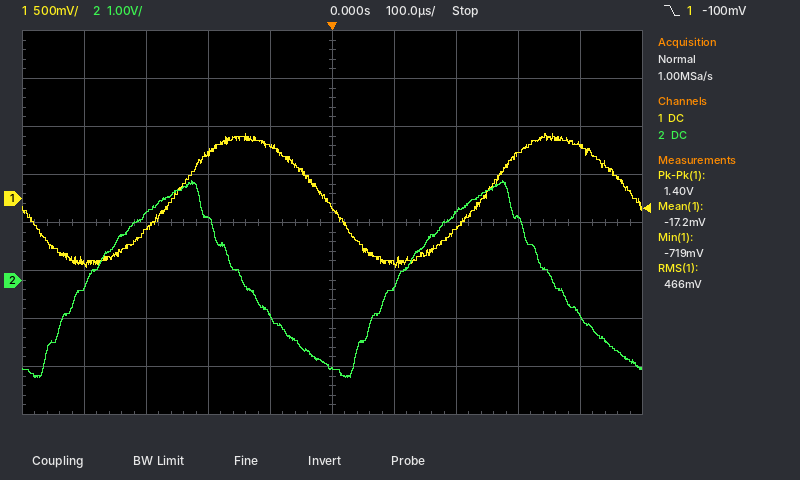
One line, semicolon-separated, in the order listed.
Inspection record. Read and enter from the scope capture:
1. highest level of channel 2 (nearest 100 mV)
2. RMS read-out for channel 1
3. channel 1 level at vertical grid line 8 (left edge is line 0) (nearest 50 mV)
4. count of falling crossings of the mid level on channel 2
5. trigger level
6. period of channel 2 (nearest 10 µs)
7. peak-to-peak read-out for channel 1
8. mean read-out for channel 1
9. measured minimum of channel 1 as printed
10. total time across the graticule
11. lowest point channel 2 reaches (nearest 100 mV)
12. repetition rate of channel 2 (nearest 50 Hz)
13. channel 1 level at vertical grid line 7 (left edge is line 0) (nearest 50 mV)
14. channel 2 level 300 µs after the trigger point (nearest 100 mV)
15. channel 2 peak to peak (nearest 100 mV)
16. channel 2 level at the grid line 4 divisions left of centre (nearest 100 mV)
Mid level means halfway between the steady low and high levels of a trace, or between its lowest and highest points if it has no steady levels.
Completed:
2.1 V; 466 mV; 450 mV; 2; -100 mV; 500 µs; 1.40 V; -17.2 mV; -719 mV; 1 ms; -2.0 V; 2.00 kHz; -300 mV; 1.3 V; 4.1 V; -100 mV
